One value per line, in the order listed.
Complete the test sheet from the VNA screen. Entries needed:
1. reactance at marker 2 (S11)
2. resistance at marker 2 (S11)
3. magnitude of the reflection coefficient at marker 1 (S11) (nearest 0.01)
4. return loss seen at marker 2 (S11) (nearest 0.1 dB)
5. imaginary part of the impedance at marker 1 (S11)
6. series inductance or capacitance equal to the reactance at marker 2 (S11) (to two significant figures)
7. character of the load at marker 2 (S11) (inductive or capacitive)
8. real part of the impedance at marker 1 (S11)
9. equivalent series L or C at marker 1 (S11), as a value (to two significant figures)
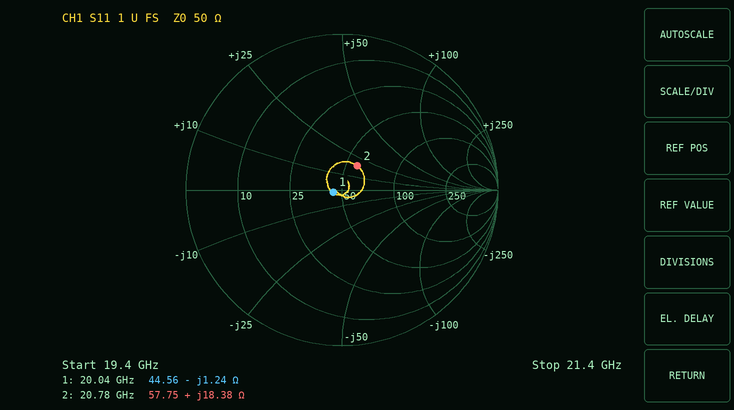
+18.38 Ω
57.75 Ω
0.06
14.8 dB
-1.24 Ω
140 pH
inductive
44.56 Ω
6.4 pF
